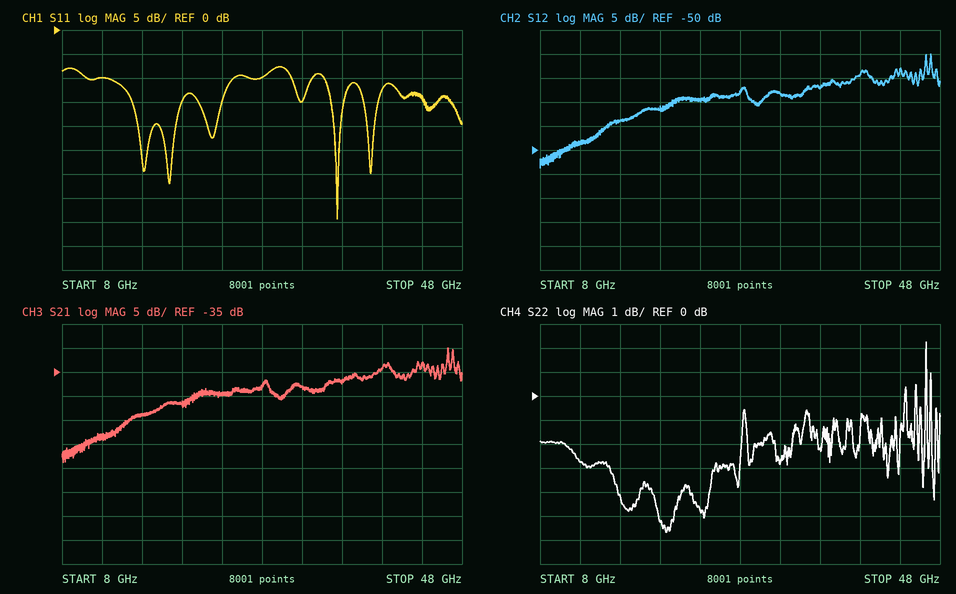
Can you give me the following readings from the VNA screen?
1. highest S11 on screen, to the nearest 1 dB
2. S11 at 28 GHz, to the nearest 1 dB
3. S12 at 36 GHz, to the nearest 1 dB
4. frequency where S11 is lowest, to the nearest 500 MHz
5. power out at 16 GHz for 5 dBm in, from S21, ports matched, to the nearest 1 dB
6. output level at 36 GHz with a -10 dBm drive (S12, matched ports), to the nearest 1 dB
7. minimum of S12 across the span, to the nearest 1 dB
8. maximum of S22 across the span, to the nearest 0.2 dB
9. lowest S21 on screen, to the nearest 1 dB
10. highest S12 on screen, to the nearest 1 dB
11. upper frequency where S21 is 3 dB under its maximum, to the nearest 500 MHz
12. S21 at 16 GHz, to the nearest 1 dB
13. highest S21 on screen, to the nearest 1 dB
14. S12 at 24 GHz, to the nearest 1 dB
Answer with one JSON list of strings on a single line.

["-8 dB", "-10 dB", "-37 dB", "35.5 GHz", "-39 dBm", "-47 dBm", "-54 dB", "2.2 dB", "-54 dB", "-30 dB", "46.5 GHz", "-44 dB", "-30 dB", "-40 dB"]
